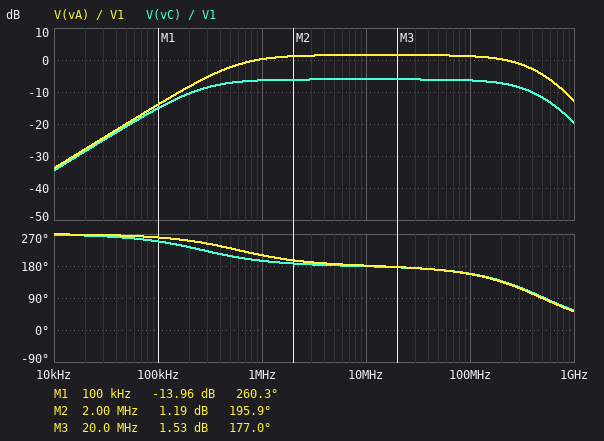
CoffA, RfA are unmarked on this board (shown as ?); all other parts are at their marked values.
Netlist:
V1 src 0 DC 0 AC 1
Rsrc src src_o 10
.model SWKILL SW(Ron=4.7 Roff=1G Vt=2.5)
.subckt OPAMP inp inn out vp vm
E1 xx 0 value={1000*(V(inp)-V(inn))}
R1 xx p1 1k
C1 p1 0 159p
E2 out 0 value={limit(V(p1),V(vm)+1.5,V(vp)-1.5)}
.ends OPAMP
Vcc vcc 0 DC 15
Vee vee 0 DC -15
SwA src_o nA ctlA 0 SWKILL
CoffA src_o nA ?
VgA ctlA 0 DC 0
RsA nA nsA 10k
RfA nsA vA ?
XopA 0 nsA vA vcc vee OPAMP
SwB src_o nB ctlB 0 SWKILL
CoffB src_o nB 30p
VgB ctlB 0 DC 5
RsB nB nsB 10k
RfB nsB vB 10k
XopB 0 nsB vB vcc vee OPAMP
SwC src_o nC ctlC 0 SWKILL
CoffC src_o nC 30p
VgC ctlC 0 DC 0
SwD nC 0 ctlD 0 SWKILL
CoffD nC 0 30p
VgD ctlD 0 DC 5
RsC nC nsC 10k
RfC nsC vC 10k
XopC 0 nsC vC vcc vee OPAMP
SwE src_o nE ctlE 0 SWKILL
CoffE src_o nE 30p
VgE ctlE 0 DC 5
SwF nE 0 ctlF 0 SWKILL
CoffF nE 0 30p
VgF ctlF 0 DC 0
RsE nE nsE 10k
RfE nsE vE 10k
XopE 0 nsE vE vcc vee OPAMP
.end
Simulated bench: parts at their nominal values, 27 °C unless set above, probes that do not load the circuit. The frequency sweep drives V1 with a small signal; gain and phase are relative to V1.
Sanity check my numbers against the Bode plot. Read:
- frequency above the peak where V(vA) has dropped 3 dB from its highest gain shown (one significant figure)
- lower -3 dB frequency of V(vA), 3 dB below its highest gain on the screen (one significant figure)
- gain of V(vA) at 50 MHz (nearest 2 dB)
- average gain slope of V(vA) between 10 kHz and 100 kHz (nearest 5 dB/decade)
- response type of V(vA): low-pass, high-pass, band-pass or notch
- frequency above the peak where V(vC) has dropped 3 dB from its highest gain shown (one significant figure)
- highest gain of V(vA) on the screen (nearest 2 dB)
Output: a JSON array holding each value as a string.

["300 MHz", "600 kHz", "2 dB", "20 dB/decade", "band-pass", "300 MHz", "2 dB"]
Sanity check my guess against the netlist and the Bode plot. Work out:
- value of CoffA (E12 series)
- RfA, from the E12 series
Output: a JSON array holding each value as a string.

["27 pF", "12 kΩ"]
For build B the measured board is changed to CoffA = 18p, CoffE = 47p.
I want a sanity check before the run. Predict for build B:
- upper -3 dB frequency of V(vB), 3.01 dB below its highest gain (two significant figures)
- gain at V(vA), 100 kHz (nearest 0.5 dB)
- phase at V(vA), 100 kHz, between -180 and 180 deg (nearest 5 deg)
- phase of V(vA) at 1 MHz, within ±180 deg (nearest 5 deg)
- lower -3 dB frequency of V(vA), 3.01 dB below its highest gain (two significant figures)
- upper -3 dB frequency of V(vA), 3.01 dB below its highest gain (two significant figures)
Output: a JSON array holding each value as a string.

["320 MHz", "-17.5 dB", "-95 deg", "-140 deg", "880 kHz", "300 MHz"]
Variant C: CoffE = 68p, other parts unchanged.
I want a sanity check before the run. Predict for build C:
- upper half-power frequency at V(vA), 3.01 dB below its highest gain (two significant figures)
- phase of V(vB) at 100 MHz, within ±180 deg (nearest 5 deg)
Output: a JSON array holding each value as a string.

["290 MHz", "155 deg"]
